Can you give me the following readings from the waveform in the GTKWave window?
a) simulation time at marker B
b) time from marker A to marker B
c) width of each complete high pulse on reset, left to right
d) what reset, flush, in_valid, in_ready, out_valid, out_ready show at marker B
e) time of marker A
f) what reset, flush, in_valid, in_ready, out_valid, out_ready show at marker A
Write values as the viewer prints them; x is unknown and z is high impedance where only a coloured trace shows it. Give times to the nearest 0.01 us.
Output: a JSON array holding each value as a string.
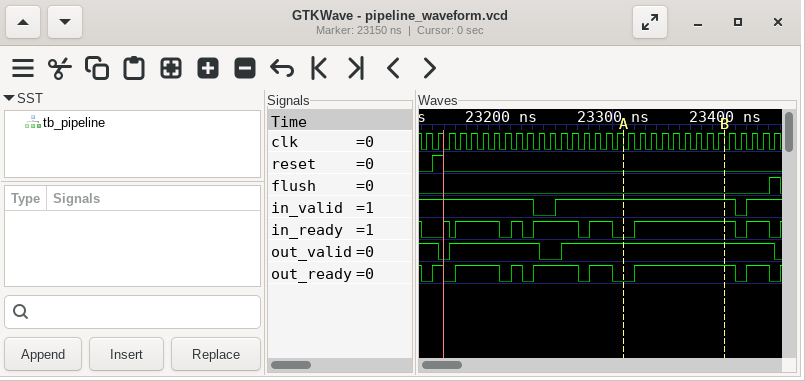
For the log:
["23.4 us", "0.09 us", "0.01 us", "reset=0, flush=0, in_valid=1, in_ready=1, out_valid=1, out_ready=1", "23.31 us", "reset=0, flush=0, in_valid=1, in_ready=0, out_valid=1, out_ready=0"]
